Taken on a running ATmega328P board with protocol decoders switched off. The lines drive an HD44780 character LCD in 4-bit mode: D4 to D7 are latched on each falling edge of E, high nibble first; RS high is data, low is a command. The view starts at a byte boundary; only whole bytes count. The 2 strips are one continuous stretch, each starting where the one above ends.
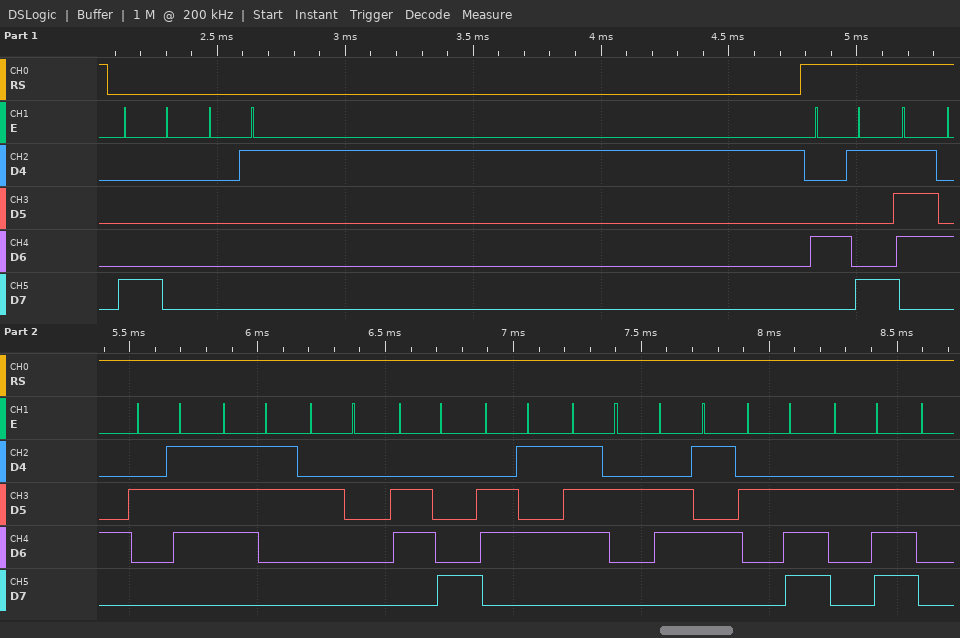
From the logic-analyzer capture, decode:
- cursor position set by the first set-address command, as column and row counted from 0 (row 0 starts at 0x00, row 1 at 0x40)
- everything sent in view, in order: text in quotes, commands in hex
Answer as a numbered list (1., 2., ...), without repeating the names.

1. column 0, row 0
2. 0x80 0x01 "It's here.."
